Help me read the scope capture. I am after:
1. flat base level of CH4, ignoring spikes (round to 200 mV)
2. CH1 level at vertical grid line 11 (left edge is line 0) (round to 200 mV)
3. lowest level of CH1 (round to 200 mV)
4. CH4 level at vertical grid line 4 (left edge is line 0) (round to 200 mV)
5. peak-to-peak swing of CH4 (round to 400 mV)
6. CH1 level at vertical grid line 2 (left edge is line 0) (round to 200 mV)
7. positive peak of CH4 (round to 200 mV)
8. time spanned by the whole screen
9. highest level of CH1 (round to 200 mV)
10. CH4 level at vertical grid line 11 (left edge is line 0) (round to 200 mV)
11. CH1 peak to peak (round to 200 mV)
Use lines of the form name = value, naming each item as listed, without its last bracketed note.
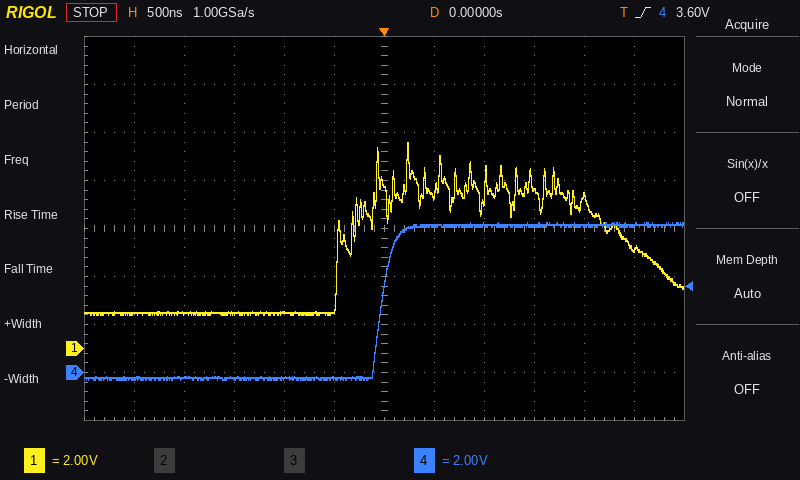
flat base level of CH4, ignoring spikes = -200 mV
CH1 level at vertical grid line 11 (left edge is line 0) = 4.2 V
lowest level of CH1 = 1.4 V
CH4 level at vertical grid line 4 (left edge is line 0) = -200 mV
peak-to-peak swing of CH4 = 6.4 V
CH1 level at vertical grid line 2 (left edge is line 0) = 1.4 V
positive peak of CH4 = 6.2 V
time spanned by the whole screen = 6 µs
highest level of CH1 = 8.6 V
CH4 level at vertical grid line 11 (left edge is line 0) = 6.2 V
CH1 peak to peak = 7.2 V
